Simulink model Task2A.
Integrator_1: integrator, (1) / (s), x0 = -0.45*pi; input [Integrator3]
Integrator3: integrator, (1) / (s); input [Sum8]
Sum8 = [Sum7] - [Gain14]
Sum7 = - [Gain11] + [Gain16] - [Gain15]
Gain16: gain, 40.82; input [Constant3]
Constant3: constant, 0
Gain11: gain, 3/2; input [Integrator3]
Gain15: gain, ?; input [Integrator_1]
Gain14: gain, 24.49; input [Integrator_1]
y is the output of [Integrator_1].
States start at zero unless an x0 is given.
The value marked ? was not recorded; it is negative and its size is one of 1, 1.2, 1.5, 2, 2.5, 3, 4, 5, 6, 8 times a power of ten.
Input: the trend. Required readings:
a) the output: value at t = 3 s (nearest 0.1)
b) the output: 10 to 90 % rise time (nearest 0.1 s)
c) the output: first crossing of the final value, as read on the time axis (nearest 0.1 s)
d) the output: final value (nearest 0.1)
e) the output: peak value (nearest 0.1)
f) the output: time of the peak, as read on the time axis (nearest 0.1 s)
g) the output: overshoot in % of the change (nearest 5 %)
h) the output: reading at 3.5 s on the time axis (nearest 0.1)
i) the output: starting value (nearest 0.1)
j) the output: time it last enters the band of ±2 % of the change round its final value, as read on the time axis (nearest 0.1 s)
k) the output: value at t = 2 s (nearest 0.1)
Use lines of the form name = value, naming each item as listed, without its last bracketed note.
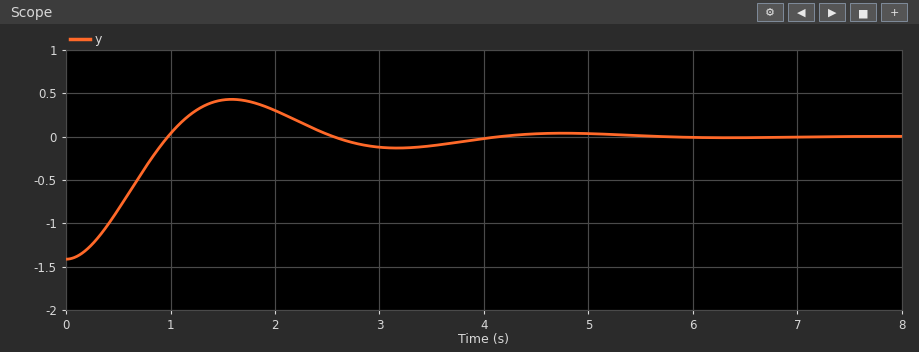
the output: value at t = 3 s = -0.1
the output: 10 to 90 % rise time = 0.7 s
the output: first crossing of the final value, as read on the time axis = 1.0 s
the output: final value = 0.0
the output: peak value = 0.4
the output: time of the peak, as read on the time axis = 1.6 s
the output: overshoot in % of the change = 30 %
the output: reading at 3.5 s on the time axis = -0.1
the output: starting value = -1.4
the output: time it last enters the band of ±2 % of the change round its final value, as read on the time axis = 5.2 s
the output: value at t = 2 s = 0.3
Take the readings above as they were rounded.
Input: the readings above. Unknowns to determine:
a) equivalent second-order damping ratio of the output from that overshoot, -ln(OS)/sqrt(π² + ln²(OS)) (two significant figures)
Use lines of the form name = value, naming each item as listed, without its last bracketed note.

equivalent second-order damping ratio of the output from that overshoot, -ln(OS)/sqrt(π² + ln²(OS)) = 0.36
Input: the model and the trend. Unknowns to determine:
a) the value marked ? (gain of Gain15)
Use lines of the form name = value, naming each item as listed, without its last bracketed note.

the value marked ? = -20
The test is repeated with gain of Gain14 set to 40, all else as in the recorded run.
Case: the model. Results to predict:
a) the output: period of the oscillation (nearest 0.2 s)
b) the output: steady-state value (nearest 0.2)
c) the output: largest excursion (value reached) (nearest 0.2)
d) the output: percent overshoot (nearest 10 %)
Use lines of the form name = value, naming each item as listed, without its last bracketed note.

the output: period of the oscillation = 1.4 s
the output: steady-state value = 0.0
the output: largest excursion (value reached) = 0.8
the output: percent overshoot = 60 %
